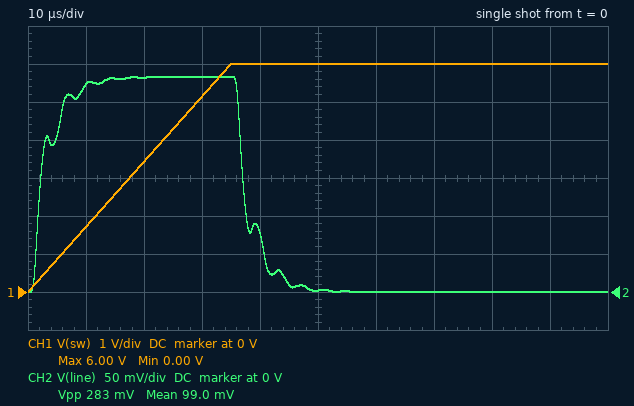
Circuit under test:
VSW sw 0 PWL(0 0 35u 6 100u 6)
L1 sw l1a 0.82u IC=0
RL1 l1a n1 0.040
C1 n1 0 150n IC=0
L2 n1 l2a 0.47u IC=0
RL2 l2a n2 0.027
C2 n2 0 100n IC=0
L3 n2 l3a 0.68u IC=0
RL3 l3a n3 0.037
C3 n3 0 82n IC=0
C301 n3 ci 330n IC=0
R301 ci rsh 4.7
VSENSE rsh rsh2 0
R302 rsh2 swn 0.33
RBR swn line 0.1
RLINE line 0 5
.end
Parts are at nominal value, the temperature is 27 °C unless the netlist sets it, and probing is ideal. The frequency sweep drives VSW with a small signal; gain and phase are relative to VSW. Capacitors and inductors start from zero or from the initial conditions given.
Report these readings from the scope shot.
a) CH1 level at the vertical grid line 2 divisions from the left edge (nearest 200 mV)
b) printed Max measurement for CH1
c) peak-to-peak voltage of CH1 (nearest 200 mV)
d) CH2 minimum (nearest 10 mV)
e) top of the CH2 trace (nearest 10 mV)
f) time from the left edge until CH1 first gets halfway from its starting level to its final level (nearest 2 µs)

3.4 V
6.00 V
6.0 V
0 V
280 mV
18 µs
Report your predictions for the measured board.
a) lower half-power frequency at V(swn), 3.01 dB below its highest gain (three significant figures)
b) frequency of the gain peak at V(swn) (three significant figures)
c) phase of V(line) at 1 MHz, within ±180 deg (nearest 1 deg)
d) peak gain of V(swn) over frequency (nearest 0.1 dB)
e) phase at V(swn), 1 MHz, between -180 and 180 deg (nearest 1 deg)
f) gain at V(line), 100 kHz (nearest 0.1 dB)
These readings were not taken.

221 kHz
264 kHz
13 deg
6.2 dB
13 deg
-5.2 dB
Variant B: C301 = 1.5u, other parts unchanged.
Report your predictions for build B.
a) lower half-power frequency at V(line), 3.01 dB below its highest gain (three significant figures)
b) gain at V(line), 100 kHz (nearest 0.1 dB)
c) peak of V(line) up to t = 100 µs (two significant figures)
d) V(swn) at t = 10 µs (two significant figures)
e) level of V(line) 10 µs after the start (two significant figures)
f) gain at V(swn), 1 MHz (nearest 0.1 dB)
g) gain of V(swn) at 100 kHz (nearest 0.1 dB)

226 kHz
-4.7 dB
1.2 V
630 mV
620 mV
-16.1 dB
-4.6 dB
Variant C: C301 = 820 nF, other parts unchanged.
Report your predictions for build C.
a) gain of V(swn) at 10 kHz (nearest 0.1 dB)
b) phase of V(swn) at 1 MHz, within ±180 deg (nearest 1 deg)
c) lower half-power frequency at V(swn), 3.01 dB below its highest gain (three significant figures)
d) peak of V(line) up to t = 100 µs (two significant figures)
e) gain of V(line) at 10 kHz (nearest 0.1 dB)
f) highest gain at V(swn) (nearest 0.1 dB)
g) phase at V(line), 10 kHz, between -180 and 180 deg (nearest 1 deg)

-12.6 dB
12 deg
224 kHz
690 mV
-12.8 dB
6.1 dB
62 deg
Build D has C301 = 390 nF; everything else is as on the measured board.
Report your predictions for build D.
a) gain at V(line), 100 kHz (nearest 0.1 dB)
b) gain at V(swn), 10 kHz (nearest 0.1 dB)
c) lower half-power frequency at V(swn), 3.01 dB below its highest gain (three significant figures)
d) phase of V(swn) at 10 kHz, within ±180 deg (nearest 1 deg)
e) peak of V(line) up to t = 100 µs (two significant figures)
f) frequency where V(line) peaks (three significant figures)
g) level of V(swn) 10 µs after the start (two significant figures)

-5.0 dB
-18.3 dB
222 kHz
76 deg
330 mV
265 kHz
320 mV
